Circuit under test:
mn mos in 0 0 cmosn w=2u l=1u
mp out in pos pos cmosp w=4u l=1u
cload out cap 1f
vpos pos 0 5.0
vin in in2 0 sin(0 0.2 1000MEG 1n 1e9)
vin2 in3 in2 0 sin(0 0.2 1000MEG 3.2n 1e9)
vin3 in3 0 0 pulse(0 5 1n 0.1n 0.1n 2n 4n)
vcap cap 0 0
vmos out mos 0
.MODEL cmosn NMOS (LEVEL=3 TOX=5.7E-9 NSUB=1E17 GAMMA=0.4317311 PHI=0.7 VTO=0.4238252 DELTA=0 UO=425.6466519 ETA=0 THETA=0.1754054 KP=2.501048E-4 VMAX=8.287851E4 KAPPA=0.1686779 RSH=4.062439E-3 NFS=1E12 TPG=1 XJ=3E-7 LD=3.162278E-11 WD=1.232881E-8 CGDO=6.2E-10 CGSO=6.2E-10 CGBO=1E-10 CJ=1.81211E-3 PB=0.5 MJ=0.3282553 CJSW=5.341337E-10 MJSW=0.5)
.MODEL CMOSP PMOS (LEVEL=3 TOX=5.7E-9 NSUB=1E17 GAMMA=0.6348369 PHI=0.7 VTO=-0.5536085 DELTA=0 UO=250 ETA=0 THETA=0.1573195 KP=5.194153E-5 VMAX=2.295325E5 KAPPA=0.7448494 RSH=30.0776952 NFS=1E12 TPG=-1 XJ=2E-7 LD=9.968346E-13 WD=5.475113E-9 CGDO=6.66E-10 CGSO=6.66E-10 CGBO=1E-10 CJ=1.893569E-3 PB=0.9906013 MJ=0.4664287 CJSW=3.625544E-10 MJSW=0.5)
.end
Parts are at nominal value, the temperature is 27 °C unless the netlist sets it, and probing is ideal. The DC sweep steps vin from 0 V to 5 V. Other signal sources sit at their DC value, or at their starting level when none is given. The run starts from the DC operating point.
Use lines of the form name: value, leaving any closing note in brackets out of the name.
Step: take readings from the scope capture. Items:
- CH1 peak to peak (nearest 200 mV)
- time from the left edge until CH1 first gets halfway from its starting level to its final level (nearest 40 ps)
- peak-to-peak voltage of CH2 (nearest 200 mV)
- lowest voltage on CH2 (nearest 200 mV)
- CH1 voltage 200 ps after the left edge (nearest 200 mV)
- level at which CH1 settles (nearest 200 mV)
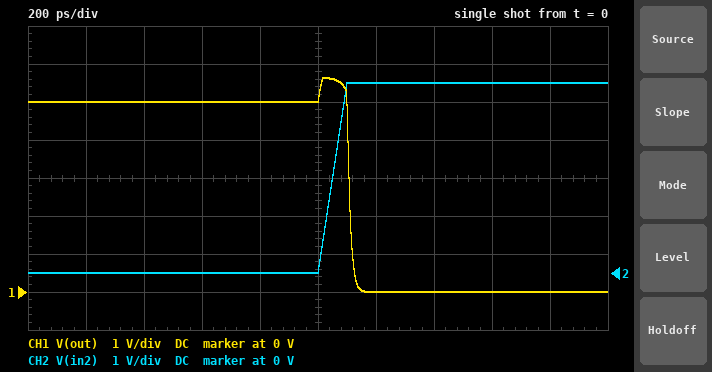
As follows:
CH1 peak to peak: 5.6 V
time from the left edge until CH1 first gets halfway from its starting level to its final level: 1.12 ns
peak-to-peak voltage of CH2: 5.0 V
lowest voltage on CH2: 0 V
CH1 voltage 200 ps after the left edge: 5.0 V
level at which CH1 settles: 0 V
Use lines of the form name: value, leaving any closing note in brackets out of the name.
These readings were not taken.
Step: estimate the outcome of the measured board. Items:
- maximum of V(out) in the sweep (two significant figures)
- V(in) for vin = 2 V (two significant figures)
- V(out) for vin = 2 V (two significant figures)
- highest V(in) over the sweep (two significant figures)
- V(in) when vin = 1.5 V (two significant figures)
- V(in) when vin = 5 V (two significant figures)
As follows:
maximum of V(out) in the sweep: 5.0 V
V(in) for vin = 2 V: 2.0 V
V(out) for vin = 2 V: 3.6 V
highest V(in) over the sweep: 5.0 V
V(in) when vin = 1.5 V: 1.5 V
V(in) when vin = 5 V: 5.0 V
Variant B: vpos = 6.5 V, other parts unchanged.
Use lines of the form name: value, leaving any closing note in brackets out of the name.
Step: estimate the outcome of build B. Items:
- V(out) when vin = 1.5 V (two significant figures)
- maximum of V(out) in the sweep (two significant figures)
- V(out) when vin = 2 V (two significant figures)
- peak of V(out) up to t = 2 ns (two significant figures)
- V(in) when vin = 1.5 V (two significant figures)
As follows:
V(out) when vin = 1.5 V: 6.1 V
maximum of V(out) in the sweep: 6.5 V
V(out) when vin = 2 V: 5.7 V
peak of V(out) up to t = 2 ns: 7.1 V
V(in) when vin = 1.5 V: 1.5 V
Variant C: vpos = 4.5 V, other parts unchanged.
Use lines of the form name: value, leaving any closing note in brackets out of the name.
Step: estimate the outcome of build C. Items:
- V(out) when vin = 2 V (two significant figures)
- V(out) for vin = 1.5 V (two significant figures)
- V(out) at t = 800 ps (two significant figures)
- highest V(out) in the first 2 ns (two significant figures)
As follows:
V(out) when vin = 2 V: 600 mV
V(out) for vin = 1.5 V: 3.9 V
V(out) at t = 800 ps: 4.5 V
highest V(out) in the first 2 ns: 5.1 V
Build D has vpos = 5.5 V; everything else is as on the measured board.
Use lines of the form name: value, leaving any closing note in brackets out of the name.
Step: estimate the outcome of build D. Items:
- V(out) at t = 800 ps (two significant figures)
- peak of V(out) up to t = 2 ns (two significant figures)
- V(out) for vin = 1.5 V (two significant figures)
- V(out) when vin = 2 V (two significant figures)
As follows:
V(out) at t = 800 ps: 5.5 V
peak of V(out) up to t = 2 ns: 6.1 V
V(out) for vin = 1.5 V: 5.1 V
V(out) when vin = 2 V: 4.5 V
